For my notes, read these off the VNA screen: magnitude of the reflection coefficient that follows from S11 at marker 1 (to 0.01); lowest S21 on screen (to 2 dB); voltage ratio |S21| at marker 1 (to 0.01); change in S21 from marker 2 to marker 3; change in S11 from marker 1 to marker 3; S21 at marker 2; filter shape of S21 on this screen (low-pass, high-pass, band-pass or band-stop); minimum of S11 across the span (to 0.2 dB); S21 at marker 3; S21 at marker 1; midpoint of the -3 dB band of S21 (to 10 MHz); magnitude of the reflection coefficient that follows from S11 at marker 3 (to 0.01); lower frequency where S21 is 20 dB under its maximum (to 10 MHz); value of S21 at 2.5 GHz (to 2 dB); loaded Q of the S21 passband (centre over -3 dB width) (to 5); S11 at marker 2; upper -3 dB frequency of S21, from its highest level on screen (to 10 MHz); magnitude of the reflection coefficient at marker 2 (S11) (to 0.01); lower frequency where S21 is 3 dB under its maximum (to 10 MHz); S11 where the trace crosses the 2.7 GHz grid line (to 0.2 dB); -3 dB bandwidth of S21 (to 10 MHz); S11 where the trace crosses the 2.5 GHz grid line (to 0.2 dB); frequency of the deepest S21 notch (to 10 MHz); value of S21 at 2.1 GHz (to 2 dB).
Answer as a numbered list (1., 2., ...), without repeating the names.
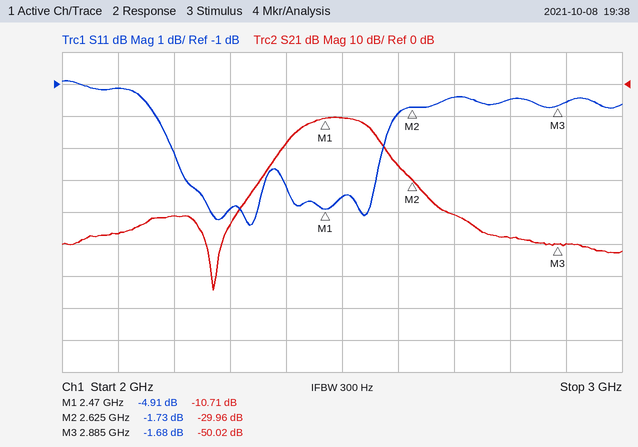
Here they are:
1. 0.57
2. -64 dB
3. 0.29
4. -20.06 dB
5. 3.23 dB
6. -29.96 dB
7. band-pass
8. -5.4 dB
9. -50.02 dB
10. -10.71 dB
11. 2.49 GHz
12. 0.82
13. 2.35 GHz
14. -10 dB
15. 20
16. -1.73 dB
17. 2.55 GHz
18. 0.82
19. 2.43 GHz
20. -1.4 dB
21. 120 MHz
22. -4.6 dB
23. 2.27 GHz
24. -46 dB
